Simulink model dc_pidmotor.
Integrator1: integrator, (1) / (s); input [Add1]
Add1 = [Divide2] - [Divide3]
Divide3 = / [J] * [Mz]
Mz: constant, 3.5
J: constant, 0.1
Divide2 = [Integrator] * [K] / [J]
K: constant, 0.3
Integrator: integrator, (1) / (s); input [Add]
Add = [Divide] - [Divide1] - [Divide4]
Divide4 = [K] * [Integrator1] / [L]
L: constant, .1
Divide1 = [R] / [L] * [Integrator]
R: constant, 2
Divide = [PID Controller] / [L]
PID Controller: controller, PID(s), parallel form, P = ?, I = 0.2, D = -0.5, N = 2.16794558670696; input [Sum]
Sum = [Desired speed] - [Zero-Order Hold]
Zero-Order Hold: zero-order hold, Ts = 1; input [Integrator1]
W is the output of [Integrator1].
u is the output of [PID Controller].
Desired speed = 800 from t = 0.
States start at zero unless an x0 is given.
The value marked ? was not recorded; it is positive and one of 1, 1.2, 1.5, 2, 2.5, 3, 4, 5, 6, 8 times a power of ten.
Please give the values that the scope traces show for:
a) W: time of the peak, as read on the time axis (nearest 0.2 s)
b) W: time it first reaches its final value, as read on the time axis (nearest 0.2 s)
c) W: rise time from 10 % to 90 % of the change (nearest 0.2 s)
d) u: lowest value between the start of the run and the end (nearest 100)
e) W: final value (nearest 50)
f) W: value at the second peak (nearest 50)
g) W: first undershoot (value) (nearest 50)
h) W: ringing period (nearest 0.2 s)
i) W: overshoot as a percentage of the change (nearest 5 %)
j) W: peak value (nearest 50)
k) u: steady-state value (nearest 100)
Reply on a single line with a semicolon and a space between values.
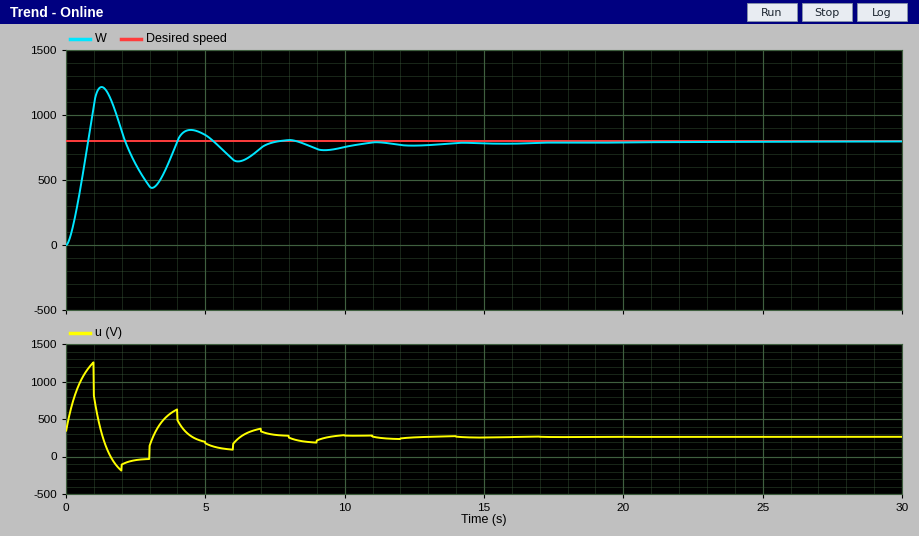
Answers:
1.2 s; 0.8 s; 0.6 s; -200; 800; 900; 450; 3.2 s; 50 %; 1200; 300
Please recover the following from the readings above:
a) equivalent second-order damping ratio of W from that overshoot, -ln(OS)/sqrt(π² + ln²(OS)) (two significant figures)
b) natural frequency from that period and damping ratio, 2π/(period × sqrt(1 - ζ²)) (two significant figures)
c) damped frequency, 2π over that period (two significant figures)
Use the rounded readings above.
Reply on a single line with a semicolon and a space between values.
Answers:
0.22; 2.0 rad/s; 2.0 rad/s
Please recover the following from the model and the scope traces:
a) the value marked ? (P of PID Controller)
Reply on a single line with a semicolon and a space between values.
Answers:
1.5
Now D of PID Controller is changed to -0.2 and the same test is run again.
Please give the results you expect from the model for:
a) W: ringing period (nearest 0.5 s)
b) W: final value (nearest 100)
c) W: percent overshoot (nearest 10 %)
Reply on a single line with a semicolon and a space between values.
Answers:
2.0 s; 800; 70 %
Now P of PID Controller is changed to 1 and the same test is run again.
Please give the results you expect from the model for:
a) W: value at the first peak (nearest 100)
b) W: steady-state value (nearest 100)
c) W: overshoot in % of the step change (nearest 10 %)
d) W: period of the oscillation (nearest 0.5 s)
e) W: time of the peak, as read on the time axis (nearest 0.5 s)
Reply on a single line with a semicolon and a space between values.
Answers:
1100; 800; 40 %; 4.0 s; 2.0 s
